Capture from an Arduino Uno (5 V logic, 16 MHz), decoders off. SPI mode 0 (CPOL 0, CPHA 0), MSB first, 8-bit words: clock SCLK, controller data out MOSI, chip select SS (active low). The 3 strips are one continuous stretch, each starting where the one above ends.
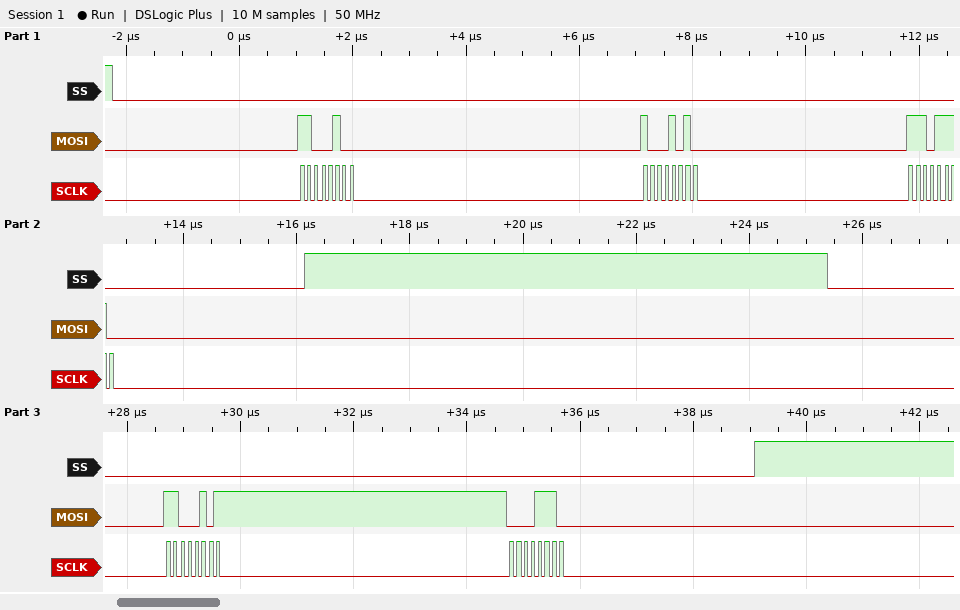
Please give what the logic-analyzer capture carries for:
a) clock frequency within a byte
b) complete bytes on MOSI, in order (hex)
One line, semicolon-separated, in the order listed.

8 MHz; C4 8A EE C5 0E
